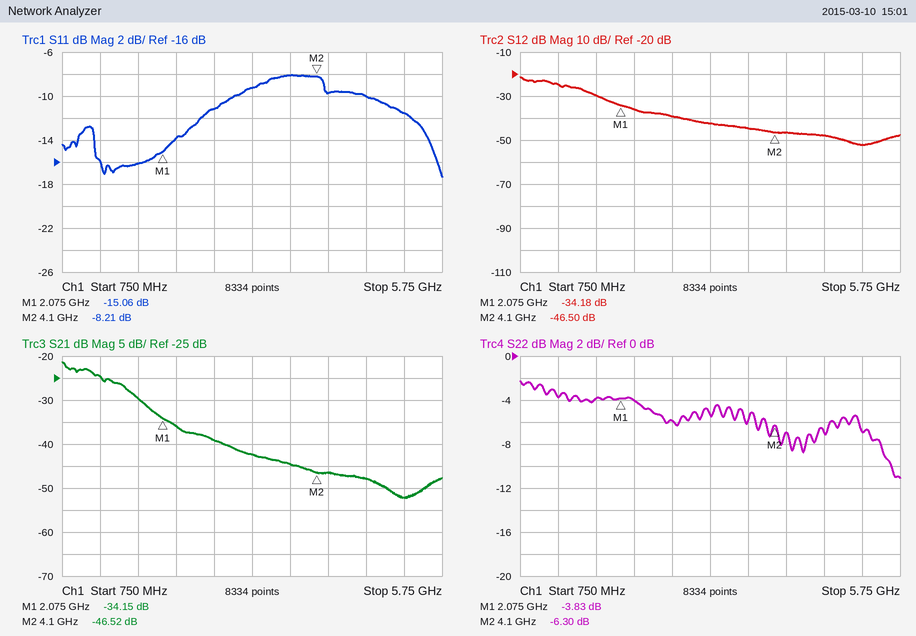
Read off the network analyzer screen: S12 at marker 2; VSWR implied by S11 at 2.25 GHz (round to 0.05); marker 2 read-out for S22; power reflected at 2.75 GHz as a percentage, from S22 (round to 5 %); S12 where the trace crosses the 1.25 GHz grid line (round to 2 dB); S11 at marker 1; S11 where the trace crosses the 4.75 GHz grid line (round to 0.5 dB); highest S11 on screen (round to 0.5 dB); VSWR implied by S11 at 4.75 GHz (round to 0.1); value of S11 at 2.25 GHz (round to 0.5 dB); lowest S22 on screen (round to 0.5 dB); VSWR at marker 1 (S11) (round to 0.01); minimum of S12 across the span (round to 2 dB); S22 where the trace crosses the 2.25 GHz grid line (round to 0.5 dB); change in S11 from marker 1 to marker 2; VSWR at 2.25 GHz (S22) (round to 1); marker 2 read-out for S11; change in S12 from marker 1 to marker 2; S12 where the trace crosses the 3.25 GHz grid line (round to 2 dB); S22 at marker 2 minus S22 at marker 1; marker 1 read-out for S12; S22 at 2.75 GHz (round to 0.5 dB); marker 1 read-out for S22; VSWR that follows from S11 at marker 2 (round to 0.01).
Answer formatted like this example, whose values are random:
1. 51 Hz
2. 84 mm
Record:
1. -46.50 dB
2. 1.50
3. -6.30 dB
4. 25 %
5. -24 dB
6. -15.06 dB
7. -10.0 dB
8. -8.0 dB
9. 1.9
10. -14.0 dB
11. -11.0 dB
12. 1.43
13. -52 dB
14. -4.0 dB
15. 6.85 dB
16. 4
17. -8.21 dB
18. -12.32 dB
19. -42 dB
20. -2.47 dB
21. -34.18 dB
22. -6.0 dB
23. -3.83 dB
24. 2.27
